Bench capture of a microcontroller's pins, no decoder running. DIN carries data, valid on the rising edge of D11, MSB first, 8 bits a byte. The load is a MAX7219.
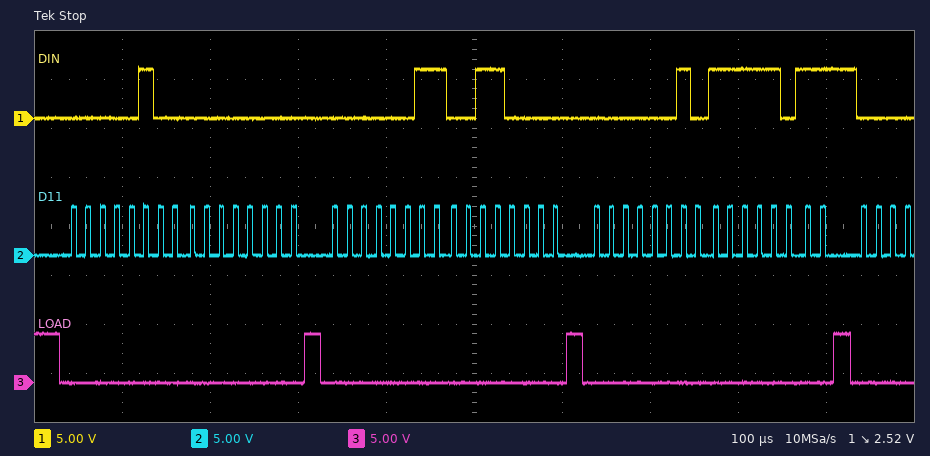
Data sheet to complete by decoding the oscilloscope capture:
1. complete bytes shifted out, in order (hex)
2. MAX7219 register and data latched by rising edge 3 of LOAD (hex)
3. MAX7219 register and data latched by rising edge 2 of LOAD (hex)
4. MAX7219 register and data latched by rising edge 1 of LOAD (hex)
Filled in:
04 00 03 30 02 FB
register 0x2, data 0xFB
register 0x3, data 0x30
register 0x4, data 0x00
